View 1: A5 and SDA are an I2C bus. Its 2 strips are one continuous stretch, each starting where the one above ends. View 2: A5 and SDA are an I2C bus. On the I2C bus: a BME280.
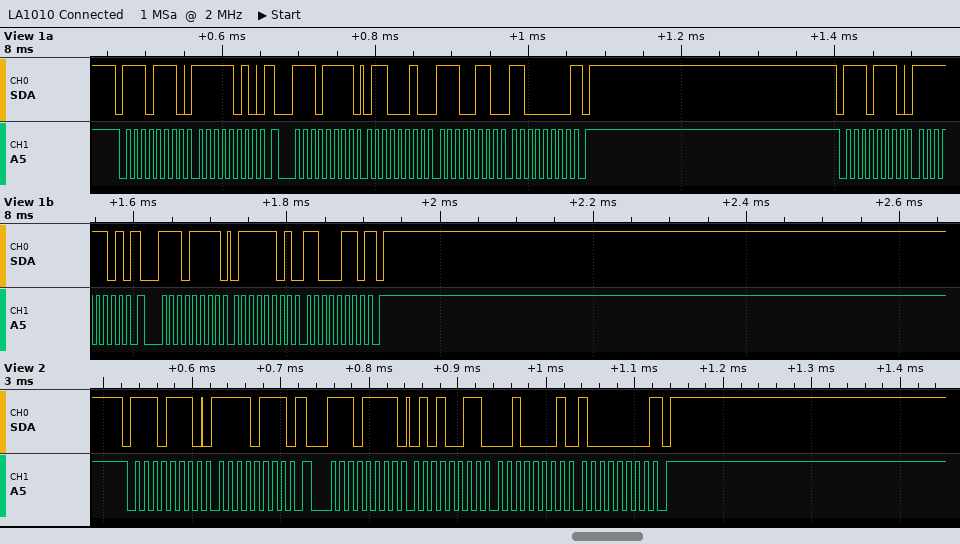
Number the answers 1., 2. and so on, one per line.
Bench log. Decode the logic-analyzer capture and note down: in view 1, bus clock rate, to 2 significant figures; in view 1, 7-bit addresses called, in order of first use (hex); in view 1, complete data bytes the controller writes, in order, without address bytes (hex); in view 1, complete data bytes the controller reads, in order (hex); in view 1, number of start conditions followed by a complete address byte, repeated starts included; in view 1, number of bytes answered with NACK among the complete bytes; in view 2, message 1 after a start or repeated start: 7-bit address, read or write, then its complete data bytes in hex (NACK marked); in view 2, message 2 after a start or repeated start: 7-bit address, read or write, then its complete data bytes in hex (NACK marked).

1. 100 kHz
2. 0x77
3. FA FD
4. 62 E6 C0 7D C6
5. 4
6. 2
7. 0x77 write: F7
8. 0x77 read: 53 21 80 NACK
